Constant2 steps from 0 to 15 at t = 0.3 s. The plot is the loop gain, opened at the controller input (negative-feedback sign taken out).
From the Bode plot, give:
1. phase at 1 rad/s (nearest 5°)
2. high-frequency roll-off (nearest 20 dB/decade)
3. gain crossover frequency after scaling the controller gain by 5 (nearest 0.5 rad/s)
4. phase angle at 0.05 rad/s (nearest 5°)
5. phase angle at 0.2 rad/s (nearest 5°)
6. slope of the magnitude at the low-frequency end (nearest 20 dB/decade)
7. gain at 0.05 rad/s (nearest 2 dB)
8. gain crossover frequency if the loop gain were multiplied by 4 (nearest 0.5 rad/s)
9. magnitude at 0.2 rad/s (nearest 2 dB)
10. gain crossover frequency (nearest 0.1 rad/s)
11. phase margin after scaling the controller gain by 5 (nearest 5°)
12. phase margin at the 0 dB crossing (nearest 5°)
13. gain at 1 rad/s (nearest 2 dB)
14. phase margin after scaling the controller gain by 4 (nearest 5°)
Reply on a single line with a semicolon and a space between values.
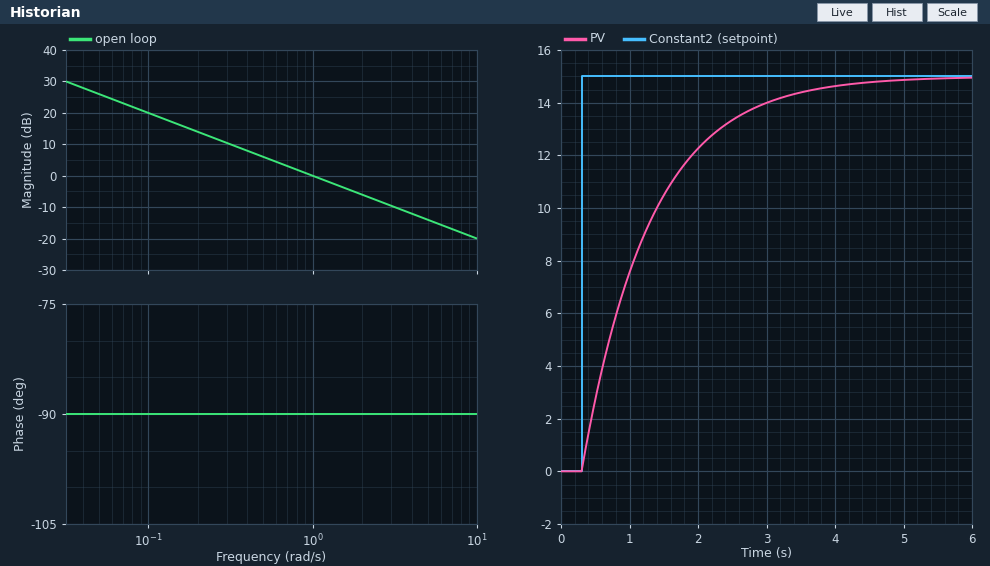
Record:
-90°; -20 dB/decade; 5.0 rad/s; -90°; -90°; -20 dB/decade; 26 dB; 4.0 rad/s; 14 dB; 1.0 rad/s; 90°; 90°; 0 dB; 90°
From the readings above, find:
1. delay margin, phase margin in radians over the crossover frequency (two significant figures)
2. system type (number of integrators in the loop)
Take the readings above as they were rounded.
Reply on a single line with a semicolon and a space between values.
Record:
1.6 s; 1
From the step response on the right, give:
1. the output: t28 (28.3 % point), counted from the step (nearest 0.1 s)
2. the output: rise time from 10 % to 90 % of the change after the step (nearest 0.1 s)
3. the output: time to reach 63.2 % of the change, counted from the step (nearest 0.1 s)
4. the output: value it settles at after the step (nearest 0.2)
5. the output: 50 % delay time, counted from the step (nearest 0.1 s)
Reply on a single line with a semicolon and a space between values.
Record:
0.3 s; 2.2 s; 1.0 s; 15.0; 0.7 s
